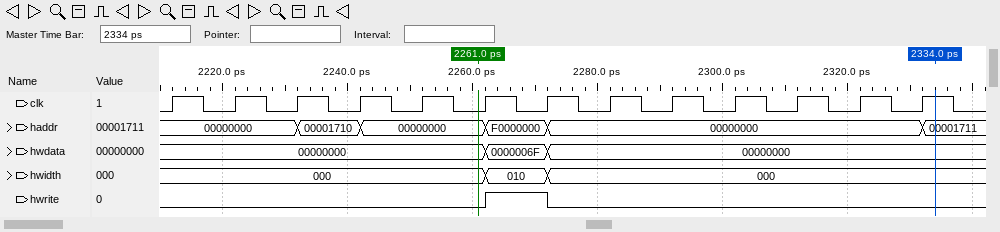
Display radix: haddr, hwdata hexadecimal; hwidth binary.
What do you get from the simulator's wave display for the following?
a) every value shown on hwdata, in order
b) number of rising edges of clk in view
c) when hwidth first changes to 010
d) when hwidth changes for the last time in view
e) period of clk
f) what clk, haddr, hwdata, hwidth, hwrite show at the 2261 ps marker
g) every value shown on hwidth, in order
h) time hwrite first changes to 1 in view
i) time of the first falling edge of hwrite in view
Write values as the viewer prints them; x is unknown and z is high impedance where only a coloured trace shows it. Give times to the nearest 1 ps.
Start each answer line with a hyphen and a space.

- 00000000, 0000006F, 00000000
- 13
- 2262 ps
- 2272 ps
- 10 ps
- clk=0, haddr=00000000, hwdata=00000000, hwidth=000, hwrite=0
- 000, 010, 000
- 2262 ps
- 2272 ps
